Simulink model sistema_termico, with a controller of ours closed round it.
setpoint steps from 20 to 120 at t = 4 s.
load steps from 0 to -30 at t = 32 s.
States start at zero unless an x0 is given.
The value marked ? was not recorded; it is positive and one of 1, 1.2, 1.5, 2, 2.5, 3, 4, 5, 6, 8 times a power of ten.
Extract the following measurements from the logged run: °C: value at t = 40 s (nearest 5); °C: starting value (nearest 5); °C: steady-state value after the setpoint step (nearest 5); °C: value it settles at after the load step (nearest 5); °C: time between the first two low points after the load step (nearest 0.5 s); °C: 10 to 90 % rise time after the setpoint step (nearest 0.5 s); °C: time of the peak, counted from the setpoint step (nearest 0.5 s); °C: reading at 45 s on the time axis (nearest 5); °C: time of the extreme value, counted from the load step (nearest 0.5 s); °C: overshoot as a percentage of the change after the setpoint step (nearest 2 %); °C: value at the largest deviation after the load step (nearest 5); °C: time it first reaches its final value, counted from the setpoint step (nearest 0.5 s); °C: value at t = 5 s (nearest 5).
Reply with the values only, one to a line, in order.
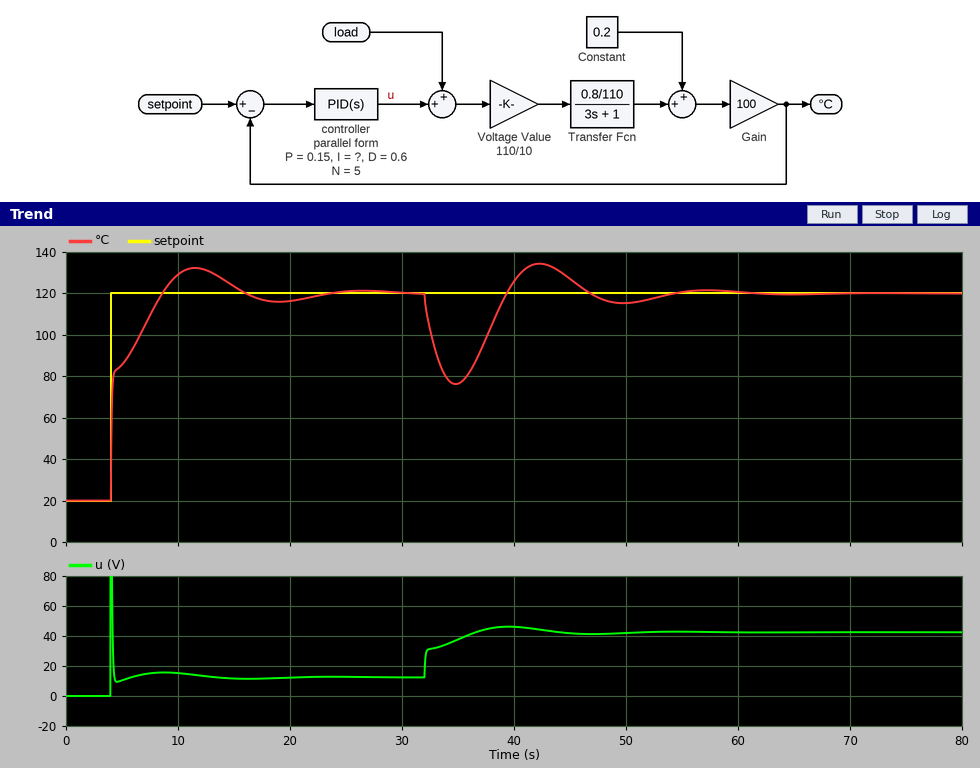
125
20
120
120
15.0 s
3.5 s
7.5 s
125
3.0 s
12 %
75
4.5 s
85
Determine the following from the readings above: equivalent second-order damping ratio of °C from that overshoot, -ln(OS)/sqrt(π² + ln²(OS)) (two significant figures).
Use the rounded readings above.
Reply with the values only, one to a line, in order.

0.56
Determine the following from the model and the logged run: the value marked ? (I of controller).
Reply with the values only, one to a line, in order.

0.2
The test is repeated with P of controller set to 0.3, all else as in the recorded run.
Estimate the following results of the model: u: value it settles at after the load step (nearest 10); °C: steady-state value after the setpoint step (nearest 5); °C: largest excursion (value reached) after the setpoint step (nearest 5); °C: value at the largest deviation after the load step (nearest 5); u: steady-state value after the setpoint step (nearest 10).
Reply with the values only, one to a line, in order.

40
120
125
85
10
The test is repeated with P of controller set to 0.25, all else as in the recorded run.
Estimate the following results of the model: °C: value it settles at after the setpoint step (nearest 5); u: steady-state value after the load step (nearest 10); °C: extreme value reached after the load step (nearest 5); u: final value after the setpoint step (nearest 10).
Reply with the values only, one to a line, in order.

120
40
80
10
